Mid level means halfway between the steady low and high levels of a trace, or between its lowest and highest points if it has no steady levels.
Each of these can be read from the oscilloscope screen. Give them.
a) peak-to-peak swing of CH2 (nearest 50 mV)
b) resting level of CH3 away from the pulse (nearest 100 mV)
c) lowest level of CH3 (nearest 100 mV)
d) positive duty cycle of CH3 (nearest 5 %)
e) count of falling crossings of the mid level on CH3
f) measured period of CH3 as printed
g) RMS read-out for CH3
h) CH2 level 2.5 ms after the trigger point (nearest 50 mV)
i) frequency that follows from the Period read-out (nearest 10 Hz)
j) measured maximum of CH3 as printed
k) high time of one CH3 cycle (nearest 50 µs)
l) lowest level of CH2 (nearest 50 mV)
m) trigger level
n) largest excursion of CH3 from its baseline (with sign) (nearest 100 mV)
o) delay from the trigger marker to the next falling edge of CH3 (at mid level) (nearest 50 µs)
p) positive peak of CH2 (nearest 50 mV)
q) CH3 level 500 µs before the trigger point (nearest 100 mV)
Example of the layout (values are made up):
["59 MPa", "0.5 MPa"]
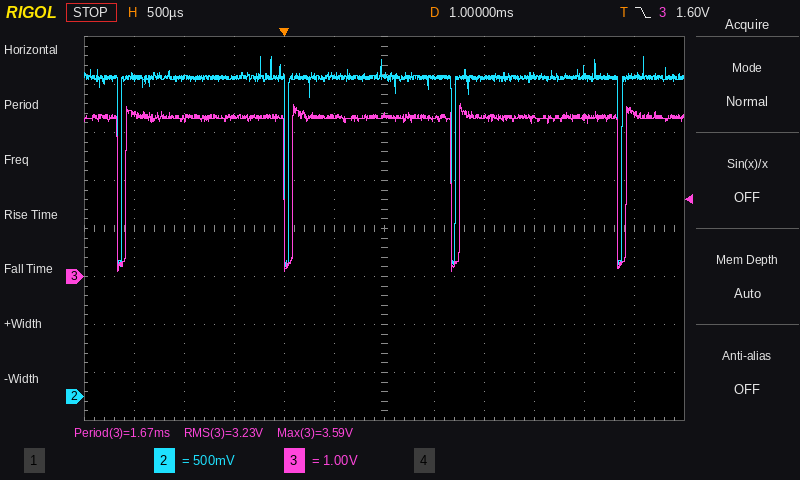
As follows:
["2.20 V", "3.3 V", "100 mV", "95 %", "4", "1.67 ms", "3.23 V", "3.35 V", "600 Hz", "3.59 V", "1.60 ms", "1.35 V", "1.60 V", "-3.2 V", "1.65 ms", "3.55 V", "3.3 V"]
